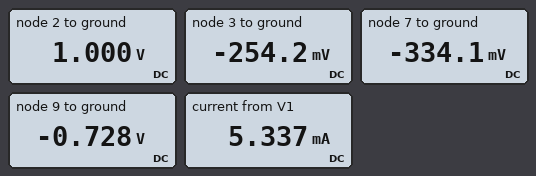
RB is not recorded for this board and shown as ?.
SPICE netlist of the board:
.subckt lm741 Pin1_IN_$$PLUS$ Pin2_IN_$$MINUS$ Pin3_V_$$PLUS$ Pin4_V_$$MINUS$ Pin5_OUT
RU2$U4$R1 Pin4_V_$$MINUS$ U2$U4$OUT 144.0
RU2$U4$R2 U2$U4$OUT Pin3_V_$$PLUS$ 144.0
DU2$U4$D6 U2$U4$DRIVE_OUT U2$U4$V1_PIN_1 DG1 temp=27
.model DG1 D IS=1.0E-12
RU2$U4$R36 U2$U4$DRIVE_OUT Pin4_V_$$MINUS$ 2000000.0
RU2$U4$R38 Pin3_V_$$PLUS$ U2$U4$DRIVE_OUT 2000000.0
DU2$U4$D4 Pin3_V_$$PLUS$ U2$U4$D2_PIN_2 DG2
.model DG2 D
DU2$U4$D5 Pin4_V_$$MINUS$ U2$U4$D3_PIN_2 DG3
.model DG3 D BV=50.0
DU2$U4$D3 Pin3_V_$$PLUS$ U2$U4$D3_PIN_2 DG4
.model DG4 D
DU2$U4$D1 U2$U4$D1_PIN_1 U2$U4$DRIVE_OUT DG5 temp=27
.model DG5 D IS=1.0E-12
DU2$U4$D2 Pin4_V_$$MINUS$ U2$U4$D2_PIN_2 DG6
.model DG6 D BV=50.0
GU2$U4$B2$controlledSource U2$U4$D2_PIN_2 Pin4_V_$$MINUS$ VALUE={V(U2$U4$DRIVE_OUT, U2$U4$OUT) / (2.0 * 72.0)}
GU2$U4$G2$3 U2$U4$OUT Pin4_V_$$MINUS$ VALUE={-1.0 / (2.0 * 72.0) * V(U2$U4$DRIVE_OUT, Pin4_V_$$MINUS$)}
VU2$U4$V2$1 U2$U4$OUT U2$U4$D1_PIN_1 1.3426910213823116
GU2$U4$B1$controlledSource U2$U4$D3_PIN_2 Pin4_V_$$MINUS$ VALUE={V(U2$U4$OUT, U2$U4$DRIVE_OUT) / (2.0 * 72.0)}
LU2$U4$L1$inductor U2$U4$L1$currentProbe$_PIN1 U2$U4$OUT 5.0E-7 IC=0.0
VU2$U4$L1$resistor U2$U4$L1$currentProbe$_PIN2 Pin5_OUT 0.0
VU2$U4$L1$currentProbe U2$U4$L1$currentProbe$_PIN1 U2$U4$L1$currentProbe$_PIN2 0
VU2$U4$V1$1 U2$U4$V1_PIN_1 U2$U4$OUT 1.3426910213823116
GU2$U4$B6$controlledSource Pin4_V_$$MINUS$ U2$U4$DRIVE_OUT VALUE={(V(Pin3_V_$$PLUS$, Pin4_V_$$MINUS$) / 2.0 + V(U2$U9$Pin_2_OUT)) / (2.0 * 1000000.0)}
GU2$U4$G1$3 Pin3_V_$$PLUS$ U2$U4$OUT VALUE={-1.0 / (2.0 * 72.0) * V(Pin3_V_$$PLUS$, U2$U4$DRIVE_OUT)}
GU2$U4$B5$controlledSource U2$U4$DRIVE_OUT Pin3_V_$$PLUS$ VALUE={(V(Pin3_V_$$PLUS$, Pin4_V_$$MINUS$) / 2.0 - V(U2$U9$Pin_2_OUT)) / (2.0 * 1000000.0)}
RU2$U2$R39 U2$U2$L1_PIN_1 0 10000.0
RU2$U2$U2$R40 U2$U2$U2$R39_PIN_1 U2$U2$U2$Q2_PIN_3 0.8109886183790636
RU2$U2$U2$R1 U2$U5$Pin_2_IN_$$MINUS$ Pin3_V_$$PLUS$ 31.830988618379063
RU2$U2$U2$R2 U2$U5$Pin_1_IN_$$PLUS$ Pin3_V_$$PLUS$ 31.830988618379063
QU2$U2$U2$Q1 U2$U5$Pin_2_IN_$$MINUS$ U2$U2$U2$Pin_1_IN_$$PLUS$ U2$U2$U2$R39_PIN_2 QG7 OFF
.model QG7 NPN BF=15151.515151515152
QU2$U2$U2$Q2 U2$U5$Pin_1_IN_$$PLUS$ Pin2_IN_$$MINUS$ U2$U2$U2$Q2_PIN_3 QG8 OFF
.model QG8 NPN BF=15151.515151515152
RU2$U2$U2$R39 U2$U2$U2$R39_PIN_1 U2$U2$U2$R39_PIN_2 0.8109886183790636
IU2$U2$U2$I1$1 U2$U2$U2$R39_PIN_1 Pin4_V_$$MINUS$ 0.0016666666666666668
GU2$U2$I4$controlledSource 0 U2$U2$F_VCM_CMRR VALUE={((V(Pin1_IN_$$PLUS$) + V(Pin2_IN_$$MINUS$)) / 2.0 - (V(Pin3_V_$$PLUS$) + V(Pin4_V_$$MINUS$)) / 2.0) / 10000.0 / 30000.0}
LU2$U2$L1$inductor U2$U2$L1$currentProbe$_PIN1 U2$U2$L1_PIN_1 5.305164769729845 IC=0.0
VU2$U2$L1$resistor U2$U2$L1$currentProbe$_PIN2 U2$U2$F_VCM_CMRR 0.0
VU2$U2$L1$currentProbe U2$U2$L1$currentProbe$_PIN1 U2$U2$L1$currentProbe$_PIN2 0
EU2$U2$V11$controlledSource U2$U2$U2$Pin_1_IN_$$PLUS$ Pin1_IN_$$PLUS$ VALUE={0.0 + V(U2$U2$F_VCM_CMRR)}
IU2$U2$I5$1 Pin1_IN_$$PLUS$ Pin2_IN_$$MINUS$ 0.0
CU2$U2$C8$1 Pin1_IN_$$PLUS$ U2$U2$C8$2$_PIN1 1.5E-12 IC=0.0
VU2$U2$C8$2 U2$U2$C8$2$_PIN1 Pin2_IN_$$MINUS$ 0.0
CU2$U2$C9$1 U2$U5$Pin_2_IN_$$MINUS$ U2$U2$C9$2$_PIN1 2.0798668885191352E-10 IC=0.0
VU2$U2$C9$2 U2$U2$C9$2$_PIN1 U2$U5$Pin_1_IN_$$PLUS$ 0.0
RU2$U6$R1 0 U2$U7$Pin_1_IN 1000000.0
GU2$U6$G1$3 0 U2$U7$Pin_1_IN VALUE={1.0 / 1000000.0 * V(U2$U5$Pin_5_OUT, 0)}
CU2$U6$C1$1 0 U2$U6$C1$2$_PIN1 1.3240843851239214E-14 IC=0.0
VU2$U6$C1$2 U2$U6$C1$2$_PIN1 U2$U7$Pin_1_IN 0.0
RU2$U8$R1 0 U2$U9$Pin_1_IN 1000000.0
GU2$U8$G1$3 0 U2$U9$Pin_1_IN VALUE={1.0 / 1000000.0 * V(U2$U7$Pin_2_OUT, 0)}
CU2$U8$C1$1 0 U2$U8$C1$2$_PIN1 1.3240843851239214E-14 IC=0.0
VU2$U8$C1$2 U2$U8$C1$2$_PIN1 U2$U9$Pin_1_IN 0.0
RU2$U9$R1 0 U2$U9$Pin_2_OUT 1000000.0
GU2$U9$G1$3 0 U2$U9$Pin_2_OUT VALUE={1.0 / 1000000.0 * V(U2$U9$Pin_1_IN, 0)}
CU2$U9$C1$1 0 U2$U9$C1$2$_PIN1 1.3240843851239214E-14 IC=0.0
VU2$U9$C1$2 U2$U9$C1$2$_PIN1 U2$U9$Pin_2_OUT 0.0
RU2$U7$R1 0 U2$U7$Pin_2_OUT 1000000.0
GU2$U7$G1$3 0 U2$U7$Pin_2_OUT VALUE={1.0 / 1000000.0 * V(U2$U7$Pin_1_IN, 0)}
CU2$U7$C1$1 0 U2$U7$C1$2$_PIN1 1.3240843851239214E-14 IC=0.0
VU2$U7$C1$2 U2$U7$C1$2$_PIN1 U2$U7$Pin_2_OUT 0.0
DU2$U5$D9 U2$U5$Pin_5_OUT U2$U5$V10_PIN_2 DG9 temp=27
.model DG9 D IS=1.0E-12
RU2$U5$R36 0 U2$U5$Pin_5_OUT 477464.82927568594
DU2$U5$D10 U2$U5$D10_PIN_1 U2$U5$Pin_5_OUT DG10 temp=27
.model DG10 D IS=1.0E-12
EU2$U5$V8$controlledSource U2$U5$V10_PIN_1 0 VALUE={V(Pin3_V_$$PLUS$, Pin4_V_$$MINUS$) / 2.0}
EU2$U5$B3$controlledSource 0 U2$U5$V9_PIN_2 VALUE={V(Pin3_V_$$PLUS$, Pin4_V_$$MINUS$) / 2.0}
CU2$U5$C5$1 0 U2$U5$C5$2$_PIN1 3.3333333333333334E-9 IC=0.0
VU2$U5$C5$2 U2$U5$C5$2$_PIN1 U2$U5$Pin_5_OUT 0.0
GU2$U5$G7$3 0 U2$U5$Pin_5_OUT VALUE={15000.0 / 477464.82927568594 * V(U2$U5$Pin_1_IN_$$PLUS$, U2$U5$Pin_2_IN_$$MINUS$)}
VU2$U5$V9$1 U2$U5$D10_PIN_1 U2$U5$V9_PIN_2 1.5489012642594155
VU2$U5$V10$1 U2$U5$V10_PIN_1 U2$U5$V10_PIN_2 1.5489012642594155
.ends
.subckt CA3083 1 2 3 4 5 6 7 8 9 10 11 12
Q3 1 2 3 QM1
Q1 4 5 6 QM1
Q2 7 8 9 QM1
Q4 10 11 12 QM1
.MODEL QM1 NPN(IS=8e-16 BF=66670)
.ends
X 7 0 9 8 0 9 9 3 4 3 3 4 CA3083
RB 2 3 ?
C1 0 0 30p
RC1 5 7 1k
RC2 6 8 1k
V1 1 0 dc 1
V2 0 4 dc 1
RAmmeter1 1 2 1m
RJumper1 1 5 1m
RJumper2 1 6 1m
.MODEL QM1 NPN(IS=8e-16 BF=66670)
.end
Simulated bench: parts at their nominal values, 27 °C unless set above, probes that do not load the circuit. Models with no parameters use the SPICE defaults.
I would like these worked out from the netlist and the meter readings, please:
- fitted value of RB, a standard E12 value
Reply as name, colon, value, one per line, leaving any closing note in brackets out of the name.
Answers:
fitted value of RB, a standard E12 value: 470 Ω
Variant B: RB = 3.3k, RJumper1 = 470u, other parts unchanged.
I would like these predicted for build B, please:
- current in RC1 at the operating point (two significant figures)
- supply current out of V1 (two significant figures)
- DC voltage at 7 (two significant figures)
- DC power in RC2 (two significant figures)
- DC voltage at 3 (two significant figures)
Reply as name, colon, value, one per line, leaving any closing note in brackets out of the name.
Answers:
current in RC1 at the operating point: 200 µA
supply current out of V1: 790 µA
DC voltage at 7: 800 mV
DC power in RC2: 39 µW
DC voltage at 3: -300 mV
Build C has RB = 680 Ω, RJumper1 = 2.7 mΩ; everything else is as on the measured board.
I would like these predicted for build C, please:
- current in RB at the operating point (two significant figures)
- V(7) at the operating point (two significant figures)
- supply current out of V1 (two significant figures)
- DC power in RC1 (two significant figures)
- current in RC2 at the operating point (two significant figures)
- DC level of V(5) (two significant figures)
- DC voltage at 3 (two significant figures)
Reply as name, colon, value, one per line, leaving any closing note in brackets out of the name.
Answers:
current in RB at the operating point: 1.9 mA
V(7) at the operating point: 71 mV
supply current out of V1: 3.7 mA
DC power in RC1: 860 µW
current in RC2 at the operating point: 930 µA
DC level of V(5): 1.0 V
DC voltage at 3: -260 mV
